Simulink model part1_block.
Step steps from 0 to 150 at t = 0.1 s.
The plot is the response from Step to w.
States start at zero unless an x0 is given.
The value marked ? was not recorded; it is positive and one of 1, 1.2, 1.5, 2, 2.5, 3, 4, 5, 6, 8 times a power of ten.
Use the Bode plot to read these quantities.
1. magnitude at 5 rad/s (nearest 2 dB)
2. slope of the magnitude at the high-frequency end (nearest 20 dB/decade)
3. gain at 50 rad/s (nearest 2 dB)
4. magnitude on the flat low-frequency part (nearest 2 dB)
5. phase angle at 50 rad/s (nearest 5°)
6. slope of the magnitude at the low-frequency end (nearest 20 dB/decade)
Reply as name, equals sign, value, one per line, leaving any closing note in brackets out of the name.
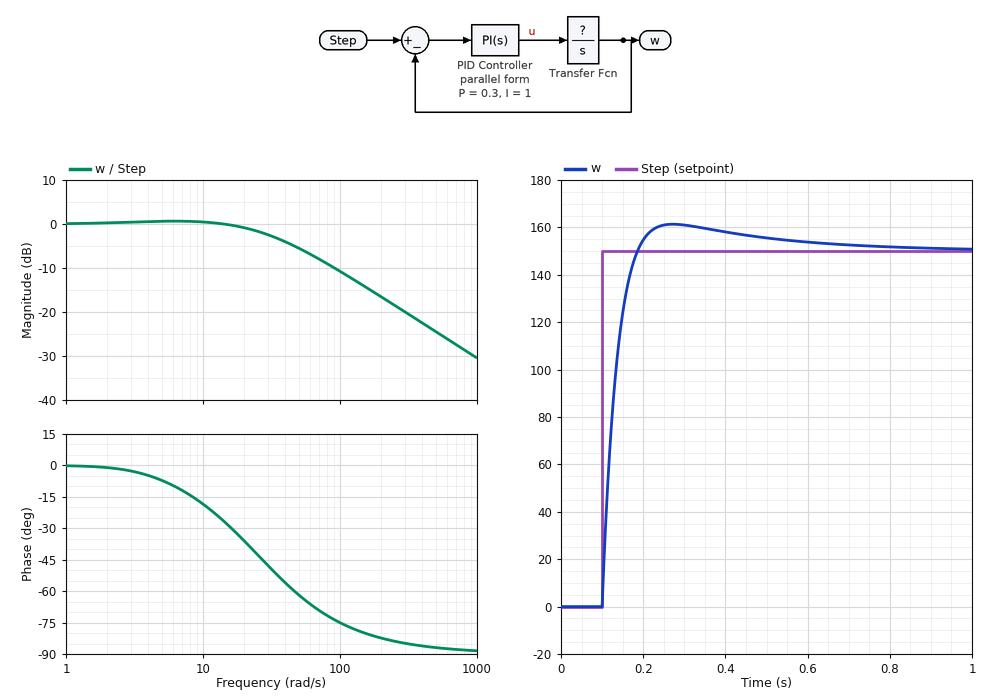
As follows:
magnitude at 5 rad/s = 0 dB
slope of the magnitude at the high-frequency end = -20 dB/decade
gain at 50 rad/s = -6 dB
magnitude on the flat low-frequency part = 0 dB
phase angle at 50 rad/s = -60°
slope of the magnitude at the low-frequency end = 0 dB/decade
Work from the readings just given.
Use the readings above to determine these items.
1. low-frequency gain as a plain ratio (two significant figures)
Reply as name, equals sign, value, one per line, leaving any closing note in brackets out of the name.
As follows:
low-frequency gain as a plain ratio = 1.0
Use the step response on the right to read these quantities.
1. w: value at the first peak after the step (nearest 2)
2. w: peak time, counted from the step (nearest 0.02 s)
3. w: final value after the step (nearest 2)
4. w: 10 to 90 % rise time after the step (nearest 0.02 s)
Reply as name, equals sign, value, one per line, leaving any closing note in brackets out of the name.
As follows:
w: value at the first peak after the step = 162
w: peak time, counted from the step = 0.18 s
w: final value after the step = 150
w: 10 to 90 % rise time after the step = 0.06 s
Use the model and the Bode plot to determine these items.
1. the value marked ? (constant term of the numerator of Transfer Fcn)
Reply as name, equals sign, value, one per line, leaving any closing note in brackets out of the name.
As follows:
the value marked ? = 100
